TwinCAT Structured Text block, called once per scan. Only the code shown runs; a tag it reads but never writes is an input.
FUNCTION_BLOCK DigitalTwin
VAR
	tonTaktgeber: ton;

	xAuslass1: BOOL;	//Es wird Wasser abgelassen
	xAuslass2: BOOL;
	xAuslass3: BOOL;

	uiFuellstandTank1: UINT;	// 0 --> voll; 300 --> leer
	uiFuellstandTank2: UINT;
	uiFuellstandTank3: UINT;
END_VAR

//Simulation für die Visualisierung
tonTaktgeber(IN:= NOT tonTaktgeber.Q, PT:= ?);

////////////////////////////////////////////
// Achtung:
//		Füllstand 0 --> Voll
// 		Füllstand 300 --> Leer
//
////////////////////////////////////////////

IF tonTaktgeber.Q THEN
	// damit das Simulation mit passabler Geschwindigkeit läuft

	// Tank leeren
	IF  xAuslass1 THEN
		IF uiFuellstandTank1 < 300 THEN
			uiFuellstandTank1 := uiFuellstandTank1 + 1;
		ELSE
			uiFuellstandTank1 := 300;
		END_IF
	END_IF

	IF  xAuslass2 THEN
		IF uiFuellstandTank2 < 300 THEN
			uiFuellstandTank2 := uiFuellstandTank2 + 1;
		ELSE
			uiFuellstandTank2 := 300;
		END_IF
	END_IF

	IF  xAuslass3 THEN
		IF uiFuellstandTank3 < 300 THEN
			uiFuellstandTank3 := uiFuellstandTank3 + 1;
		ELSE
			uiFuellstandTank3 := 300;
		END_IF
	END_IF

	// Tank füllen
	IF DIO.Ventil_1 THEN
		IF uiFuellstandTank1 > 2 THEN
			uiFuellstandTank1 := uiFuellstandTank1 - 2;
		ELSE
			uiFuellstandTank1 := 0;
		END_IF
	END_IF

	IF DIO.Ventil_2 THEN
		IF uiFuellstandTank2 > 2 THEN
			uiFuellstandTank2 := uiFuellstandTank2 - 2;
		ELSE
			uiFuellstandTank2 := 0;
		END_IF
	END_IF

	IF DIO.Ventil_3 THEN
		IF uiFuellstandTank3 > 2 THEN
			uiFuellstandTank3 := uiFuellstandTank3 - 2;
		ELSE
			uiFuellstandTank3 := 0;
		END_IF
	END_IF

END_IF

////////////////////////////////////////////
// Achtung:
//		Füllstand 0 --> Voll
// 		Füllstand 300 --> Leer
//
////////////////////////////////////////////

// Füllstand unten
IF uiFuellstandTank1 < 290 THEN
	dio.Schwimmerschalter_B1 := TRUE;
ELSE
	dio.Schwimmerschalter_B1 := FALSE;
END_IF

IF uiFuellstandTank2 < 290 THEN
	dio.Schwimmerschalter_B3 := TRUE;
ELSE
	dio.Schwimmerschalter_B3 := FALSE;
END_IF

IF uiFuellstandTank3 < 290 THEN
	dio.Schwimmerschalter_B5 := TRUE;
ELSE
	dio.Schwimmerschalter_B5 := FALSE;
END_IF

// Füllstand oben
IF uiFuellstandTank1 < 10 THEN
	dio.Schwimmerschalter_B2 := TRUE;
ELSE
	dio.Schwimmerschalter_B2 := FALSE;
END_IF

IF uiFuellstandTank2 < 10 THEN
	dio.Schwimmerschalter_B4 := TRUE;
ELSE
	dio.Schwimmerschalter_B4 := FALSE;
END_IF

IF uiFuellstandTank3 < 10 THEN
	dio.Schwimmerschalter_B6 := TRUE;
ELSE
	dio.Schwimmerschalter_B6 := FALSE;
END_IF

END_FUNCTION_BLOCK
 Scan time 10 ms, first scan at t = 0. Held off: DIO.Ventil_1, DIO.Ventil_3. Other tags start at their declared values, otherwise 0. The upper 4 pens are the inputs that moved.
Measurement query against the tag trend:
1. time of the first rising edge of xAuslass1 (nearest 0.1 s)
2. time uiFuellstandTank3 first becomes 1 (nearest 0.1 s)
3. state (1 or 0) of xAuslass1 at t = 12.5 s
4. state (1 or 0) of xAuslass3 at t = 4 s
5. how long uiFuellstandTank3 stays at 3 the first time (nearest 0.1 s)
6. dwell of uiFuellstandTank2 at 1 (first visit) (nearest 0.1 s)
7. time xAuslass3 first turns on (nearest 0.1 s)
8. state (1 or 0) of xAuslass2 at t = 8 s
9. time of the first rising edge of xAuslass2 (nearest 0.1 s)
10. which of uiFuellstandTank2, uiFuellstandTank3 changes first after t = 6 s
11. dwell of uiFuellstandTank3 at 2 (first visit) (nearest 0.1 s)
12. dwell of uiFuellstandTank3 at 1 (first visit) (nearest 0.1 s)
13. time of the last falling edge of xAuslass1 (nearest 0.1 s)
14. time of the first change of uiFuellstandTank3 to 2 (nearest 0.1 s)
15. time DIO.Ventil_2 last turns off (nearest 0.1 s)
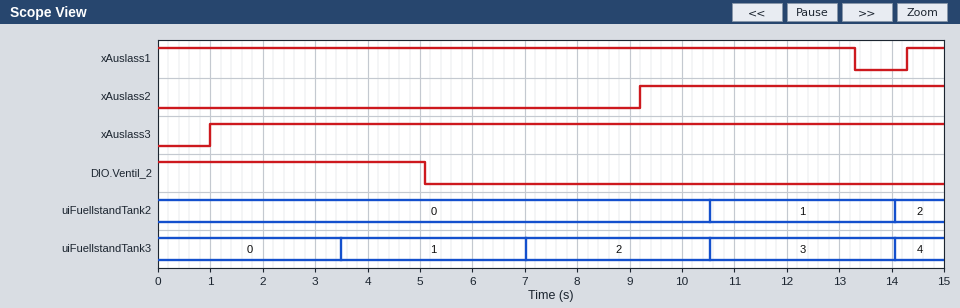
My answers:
14.3 s
3.5 s
1
1
3.5 s
3.5 s
1.0 s
0
9.2 s
uiFuellstandTank3
3.5 s
3.5 s
13.3 s
7.0 s
5.1 s
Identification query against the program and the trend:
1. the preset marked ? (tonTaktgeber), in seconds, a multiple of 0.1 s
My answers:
3.5 s
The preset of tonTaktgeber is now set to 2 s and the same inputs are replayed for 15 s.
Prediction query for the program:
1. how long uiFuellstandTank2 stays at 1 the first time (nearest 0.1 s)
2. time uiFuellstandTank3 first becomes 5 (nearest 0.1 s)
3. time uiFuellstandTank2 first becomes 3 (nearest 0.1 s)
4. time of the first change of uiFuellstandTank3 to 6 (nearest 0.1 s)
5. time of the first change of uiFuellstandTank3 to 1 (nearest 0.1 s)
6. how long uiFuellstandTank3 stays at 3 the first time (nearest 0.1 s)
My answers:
2.0 s
10.1 s
14.1 s
12.1 s
2.0 s
2.0 s
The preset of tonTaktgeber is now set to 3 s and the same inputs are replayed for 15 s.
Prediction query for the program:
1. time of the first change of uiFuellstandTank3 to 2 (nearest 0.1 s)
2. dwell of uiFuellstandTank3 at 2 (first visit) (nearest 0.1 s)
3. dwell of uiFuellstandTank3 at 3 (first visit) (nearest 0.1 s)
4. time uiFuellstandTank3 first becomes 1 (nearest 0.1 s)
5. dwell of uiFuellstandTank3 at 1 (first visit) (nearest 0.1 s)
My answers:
6.0 s
3.0 s
3.0 s
3.0 s
3.0 s
